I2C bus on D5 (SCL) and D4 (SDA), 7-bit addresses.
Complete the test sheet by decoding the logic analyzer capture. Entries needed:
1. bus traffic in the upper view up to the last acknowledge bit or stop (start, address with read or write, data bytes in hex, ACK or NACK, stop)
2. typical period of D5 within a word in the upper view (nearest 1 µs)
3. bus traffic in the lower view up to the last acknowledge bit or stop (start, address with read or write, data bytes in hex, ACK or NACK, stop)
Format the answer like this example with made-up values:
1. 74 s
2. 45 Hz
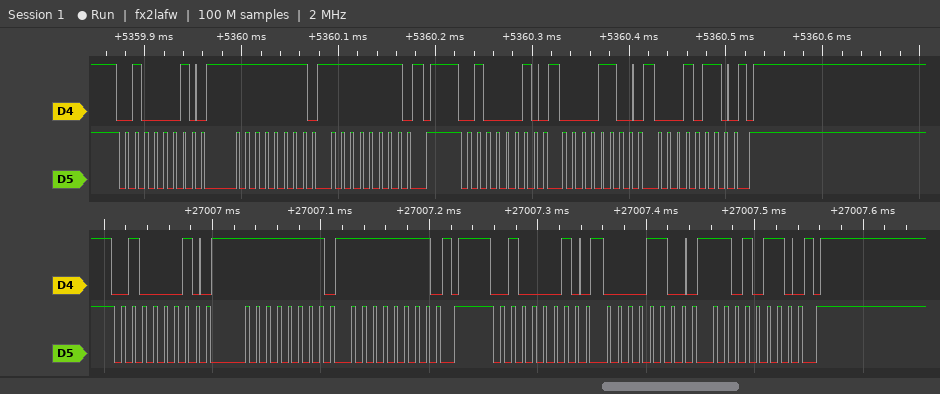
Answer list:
1. start, address 21 write ACK, FF ACK, FF ACK, stop, start, address 21 write ACK, 0C ACK, 16 ACK, stop
2. 10 µs
3. start, address 21 write ACK, FF ACK, FF ACK, stop, start, address 21 write ACK, 0C ACK, D6 ACK, stop
